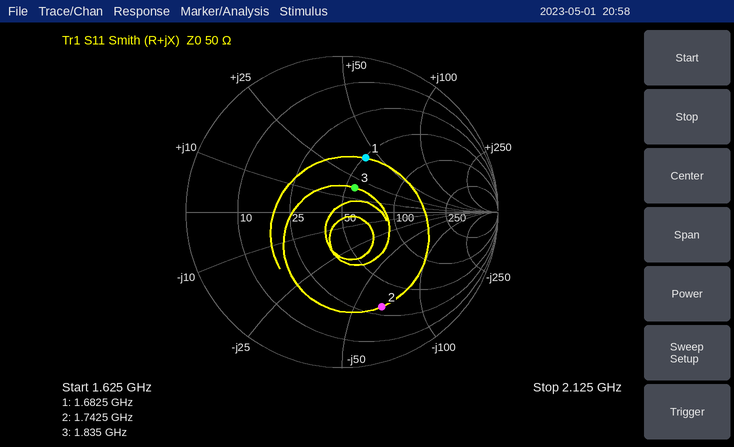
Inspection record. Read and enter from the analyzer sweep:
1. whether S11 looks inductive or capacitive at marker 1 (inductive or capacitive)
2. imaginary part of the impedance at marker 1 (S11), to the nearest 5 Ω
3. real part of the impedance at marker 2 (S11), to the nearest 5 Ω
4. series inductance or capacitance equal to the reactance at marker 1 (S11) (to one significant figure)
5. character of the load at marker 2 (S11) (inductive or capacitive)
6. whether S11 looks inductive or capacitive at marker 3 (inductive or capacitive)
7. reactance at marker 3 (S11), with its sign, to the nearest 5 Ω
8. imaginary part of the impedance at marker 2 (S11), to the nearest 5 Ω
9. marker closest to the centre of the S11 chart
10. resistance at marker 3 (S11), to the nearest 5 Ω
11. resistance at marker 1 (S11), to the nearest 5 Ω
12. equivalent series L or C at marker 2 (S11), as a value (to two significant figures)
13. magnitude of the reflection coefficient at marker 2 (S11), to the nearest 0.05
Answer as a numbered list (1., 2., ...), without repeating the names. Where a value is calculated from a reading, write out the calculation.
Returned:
1. inductive
2. +40 Ω
3. 30 Ω
4. L = 40 Ω/(2π × 1.6825 GHz) ≈ 4 nH
5. capacitive
6. inductive
7. +20 Ω
8. -65 Ω
9. marker 3
10. 55 Ω
11. 50 Ω
12. C = 1/(2π × 1.7425 GHz × 65 Ω) ≈ 1.4 pF
13. 0.65
